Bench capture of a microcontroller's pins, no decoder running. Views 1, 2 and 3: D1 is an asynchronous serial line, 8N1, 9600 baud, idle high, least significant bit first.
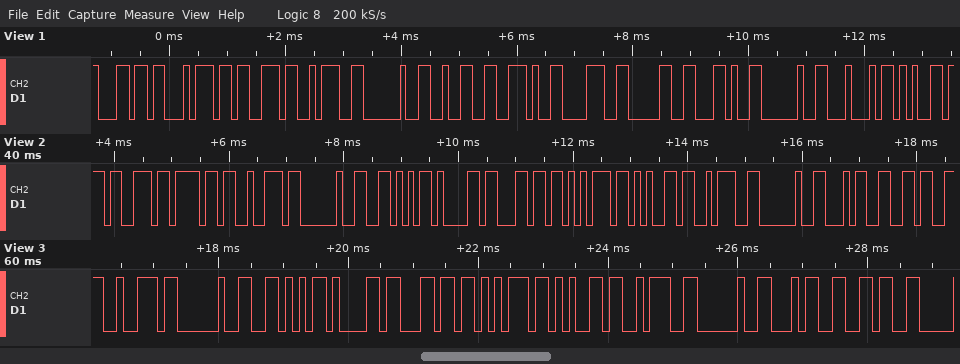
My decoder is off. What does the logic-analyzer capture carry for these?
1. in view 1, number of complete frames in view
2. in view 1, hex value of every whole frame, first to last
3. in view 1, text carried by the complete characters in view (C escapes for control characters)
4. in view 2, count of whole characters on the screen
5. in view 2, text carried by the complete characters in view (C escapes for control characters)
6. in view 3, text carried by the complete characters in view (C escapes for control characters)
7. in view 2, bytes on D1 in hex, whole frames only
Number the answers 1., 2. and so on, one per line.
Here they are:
1. 13
2. 6C 74 73 3A 20 32 2E 38 30 2C 20 44 65
3. "lts: 2.80, De"
4. 13
5. "sor Value: 46"
6. "r Value: 46"
7. 73 6F 72 20 56 61 6C 75 65 3A 20 34 36
